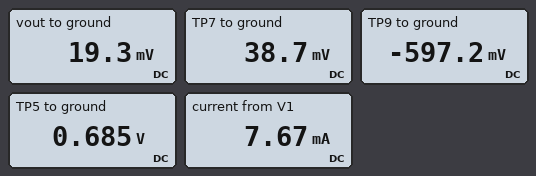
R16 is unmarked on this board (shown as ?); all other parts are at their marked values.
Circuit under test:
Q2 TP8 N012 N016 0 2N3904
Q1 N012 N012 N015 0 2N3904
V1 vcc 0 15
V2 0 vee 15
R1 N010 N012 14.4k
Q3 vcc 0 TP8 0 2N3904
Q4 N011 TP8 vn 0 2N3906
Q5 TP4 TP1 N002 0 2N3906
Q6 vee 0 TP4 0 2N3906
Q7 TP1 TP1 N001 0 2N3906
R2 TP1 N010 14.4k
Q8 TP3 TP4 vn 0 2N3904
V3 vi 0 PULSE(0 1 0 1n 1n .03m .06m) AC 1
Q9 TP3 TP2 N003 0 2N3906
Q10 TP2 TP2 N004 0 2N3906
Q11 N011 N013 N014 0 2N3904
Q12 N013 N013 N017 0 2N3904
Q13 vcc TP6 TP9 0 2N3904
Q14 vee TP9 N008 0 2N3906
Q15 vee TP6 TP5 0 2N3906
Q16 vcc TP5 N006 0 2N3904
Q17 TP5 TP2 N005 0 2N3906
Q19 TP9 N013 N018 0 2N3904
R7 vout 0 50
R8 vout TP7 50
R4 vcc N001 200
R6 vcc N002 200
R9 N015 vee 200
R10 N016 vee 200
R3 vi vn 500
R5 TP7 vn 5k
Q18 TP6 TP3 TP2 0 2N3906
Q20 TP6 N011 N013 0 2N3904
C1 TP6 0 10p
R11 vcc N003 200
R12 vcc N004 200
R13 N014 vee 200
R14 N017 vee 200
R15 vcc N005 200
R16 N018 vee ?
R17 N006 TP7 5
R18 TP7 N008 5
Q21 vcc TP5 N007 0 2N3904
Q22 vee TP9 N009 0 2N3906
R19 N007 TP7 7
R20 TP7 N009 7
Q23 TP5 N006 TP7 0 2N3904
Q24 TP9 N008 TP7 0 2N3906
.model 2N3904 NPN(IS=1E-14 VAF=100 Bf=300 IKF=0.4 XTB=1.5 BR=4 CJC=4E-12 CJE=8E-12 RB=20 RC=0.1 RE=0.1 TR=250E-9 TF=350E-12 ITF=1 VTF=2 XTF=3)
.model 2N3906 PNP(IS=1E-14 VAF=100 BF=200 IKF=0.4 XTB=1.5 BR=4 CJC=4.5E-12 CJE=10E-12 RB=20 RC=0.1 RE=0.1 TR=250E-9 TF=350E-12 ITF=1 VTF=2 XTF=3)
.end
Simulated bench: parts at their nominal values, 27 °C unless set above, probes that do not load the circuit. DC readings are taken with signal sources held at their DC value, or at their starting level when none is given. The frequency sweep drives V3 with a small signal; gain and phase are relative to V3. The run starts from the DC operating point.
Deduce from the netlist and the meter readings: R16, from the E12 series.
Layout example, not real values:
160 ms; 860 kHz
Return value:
470 Ω
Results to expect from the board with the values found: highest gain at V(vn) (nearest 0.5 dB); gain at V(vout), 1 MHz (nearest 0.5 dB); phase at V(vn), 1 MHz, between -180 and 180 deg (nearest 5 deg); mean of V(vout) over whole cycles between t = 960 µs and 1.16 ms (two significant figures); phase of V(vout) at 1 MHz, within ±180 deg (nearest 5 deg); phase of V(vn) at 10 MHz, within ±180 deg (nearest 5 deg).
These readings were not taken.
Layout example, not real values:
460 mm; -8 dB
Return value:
-27.5 dB; 12.5 dB; 60 deg; -2.4 V; 150 deg; 15 deg
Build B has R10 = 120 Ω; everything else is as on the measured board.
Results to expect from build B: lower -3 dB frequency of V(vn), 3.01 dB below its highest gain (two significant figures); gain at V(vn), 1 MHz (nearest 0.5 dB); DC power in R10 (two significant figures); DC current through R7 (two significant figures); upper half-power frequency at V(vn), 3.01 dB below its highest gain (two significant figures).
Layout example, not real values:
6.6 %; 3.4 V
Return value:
63 MHz; -39.5 dB; 290 µW; 160 µA; 2.4 GHz
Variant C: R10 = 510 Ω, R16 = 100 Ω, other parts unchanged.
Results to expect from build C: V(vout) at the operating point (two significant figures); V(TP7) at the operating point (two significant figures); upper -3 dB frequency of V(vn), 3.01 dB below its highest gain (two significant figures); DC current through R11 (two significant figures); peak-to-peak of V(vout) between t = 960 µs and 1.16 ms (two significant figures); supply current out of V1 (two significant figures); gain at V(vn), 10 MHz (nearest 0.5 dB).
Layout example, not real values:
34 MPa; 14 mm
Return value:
60 mV; 120 mV; 790 MHz; 640 µA; 5.0 V; 7.6 mA; -28.0 dB
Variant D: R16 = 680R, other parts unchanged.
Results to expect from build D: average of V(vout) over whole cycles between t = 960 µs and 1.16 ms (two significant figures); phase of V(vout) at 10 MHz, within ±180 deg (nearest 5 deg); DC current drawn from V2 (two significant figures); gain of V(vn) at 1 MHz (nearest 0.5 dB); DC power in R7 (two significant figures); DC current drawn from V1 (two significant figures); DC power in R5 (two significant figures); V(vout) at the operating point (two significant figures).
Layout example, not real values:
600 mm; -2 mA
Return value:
-2.3 V; 90 deg; 7.0 mA; -37.0 dB; 9.0 µW; 7.4 mA; 360 nW; 21 mV
